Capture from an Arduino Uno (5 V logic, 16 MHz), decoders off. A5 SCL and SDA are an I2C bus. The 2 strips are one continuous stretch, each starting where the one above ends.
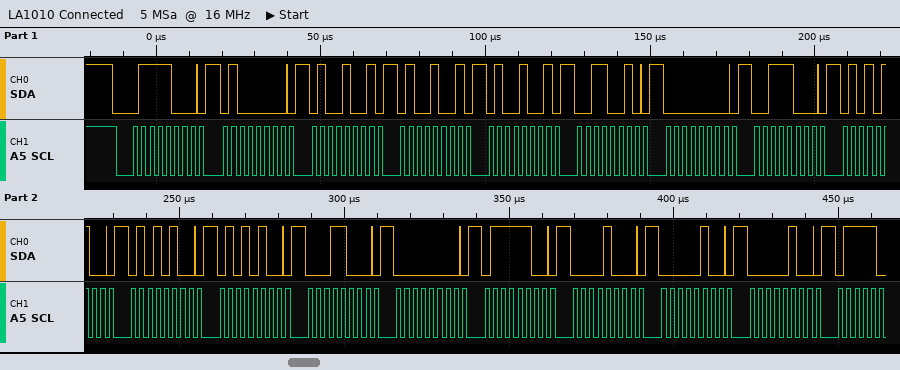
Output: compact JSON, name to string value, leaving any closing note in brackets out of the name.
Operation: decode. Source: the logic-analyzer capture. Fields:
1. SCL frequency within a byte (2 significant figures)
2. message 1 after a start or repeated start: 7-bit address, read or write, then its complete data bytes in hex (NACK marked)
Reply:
{"SCL frequency within a byte": "400 kHz", "message 1 after a start or repeated start: 7-bit address, read or write, then its complete data bytes in hex": "0x3C write: 40 49 49 49 32 00 38 54 54 54 18 00 7C 08 04 04"}
